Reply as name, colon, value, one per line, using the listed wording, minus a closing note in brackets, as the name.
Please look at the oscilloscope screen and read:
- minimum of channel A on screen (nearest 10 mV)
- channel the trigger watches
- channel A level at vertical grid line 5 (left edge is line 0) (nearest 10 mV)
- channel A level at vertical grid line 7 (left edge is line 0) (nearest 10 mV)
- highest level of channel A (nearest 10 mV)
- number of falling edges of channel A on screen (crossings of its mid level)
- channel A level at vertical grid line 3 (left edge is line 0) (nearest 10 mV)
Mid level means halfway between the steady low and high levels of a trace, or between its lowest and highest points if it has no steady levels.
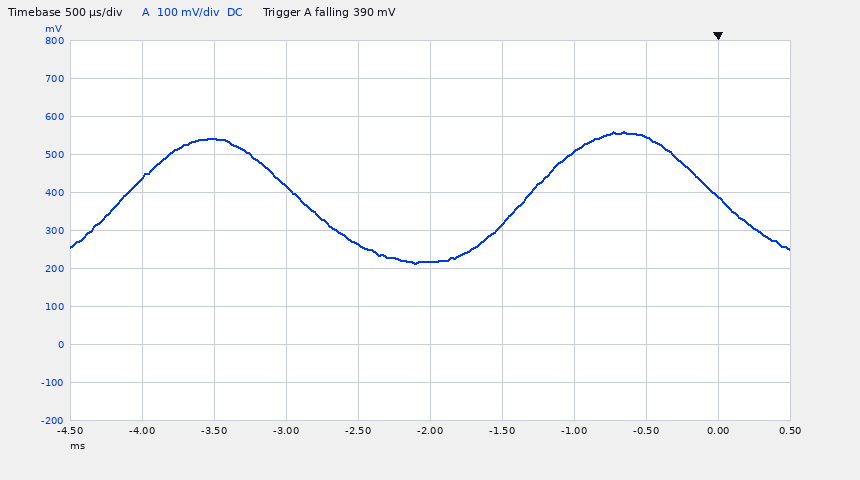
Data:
minimum of channel A on screen: 210 mV
channel the trigger watches: channel A
channel A level at vertical grid line 5 (left edge is line 0): 220 mV
channel A level at vertical grid line 7 (left edge is line 0): 510 mV
highest level of channel A: 560 mV
number of falling edges of channel A on screen: 2
channel A level at vertical grid line 3 (left edge is line 0): 420 mV
